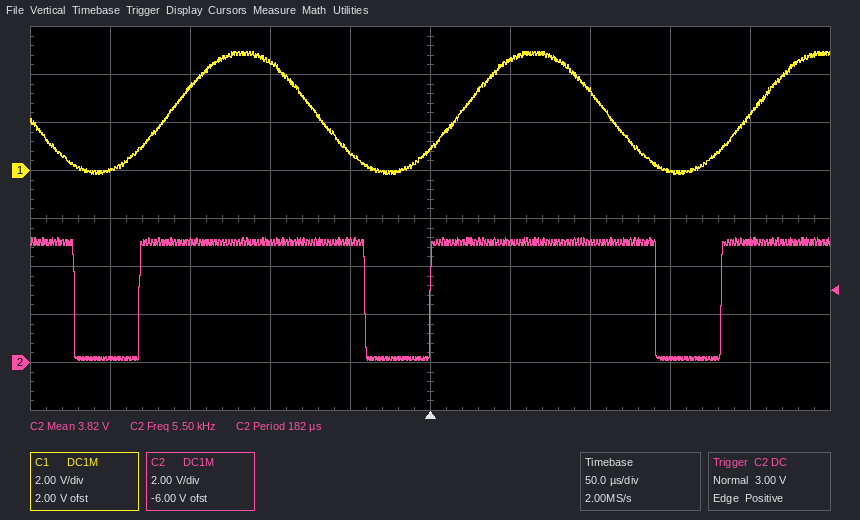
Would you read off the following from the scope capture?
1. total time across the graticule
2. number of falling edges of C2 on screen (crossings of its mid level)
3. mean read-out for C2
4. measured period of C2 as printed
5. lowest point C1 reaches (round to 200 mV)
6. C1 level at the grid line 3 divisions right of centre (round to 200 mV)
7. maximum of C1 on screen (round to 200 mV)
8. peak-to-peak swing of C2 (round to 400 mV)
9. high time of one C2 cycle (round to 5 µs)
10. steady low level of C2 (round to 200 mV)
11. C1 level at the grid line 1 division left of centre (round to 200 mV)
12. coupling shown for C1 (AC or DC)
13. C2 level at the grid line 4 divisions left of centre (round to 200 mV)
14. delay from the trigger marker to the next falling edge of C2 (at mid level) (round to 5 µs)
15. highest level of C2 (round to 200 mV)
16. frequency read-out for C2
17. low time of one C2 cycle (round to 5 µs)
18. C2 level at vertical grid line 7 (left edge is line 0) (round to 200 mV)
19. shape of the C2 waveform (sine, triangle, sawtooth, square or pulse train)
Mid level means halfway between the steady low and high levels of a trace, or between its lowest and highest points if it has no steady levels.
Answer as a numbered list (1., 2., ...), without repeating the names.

1. 500 µs
2. 3
3. 3.82 V
4. 182 µs
5. -200 mV
6. 0.0 V
7. 5.0 V
8. 5.2 V
9. 140 µs
10. 200 mV
11. 800 mV
12. DC
13. 200 mV
14. 140 µs
15. 5.2 V
16. 5.50 kHz
17. 40 µs
18. 5.0 V
19. pulse train
